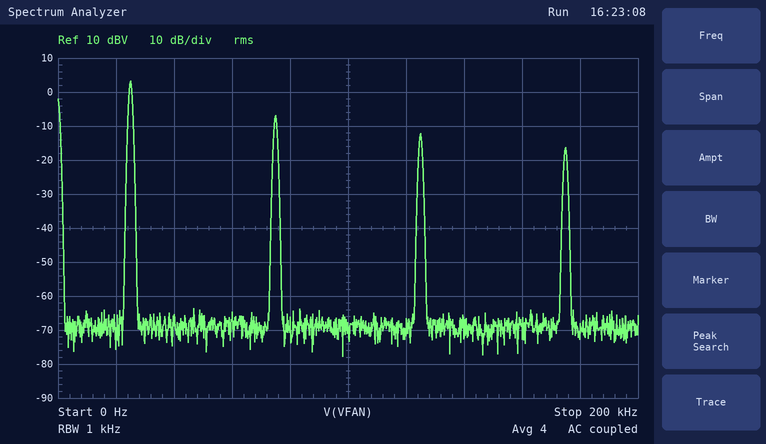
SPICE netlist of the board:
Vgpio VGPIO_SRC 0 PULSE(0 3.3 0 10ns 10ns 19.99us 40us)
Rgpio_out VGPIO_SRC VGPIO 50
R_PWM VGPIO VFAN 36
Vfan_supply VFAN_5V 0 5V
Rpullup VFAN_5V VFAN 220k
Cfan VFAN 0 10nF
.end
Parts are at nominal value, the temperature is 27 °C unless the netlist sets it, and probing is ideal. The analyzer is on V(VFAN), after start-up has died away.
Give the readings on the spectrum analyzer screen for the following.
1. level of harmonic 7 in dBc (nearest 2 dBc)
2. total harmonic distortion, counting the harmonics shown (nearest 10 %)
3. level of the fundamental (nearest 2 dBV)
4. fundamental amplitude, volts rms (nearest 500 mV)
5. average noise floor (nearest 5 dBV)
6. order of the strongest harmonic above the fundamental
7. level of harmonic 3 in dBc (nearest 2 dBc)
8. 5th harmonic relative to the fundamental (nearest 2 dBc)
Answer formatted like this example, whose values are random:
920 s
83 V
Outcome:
-20 dBc
40 %
4 dBV
1.5 V
-70 dBV
3
-10 dBc
-16 dBc
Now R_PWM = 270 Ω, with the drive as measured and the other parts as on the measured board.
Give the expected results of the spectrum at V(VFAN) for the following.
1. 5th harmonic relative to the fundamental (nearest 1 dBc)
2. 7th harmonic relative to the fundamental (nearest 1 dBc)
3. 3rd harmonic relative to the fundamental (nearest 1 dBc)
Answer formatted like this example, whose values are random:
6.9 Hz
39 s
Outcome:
-22 dBc
-27 dBc
-14 dBc
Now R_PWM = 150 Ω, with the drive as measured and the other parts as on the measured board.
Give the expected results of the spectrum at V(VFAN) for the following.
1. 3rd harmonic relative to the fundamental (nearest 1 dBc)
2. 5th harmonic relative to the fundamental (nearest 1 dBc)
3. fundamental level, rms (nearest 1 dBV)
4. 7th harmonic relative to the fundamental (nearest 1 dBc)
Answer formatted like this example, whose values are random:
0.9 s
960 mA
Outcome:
-12 dBc
-19 dBc
3 dBV
-24 dBc
